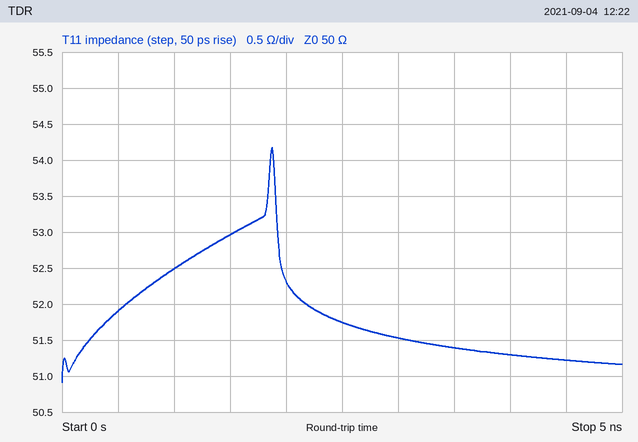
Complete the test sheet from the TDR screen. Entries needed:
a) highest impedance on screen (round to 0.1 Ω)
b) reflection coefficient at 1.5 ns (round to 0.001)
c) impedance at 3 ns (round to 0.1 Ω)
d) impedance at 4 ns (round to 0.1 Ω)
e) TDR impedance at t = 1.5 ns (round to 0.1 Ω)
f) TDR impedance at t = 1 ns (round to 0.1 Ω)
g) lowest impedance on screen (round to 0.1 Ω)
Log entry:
54.2 Ω
+0.029
51.5 Ω
51.3 Ω
53.0 Ω
52.5 Ω
50.9 Ω
